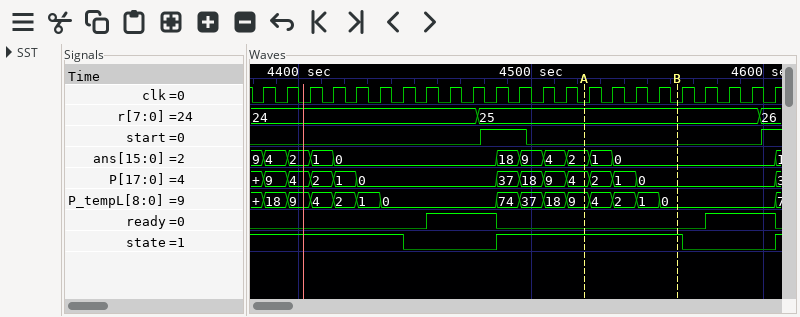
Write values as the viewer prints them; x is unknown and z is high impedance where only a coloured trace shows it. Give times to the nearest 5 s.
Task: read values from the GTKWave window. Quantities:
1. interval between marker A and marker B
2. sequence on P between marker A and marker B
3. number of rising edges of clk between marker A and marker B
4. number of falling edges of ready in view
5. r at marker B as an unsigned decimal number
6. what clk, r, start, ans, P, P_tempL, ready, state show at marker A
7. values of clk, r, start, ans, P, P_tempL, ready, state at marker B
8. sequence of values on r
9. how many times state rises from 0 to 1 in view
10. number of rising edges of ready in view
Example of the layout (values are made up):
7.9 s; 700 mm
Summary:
40 s; 4, 2, 1, 0; 4; 2; 37; clk=0, r=25, start=0, ans=2, P=4, P_tempL=9, ready=0, state=1; clk=0, r=25, start=0, ans=0, P=0, P_tempL=0, ready=0, state=1; 24, 25, 26; 2; 2
